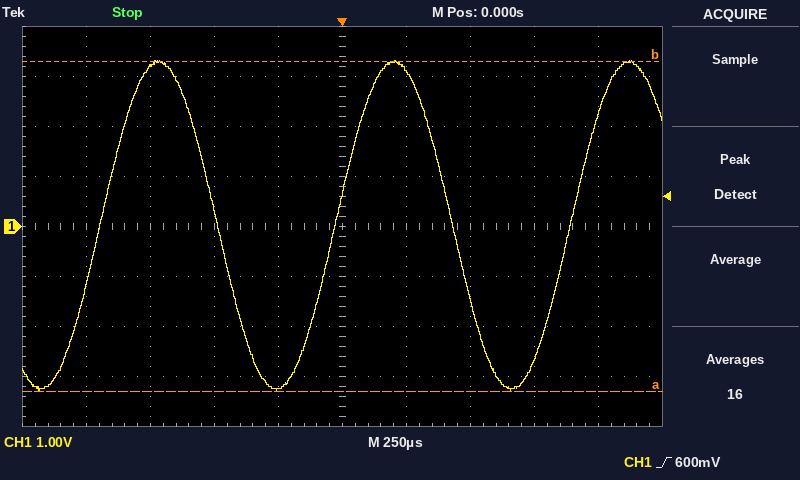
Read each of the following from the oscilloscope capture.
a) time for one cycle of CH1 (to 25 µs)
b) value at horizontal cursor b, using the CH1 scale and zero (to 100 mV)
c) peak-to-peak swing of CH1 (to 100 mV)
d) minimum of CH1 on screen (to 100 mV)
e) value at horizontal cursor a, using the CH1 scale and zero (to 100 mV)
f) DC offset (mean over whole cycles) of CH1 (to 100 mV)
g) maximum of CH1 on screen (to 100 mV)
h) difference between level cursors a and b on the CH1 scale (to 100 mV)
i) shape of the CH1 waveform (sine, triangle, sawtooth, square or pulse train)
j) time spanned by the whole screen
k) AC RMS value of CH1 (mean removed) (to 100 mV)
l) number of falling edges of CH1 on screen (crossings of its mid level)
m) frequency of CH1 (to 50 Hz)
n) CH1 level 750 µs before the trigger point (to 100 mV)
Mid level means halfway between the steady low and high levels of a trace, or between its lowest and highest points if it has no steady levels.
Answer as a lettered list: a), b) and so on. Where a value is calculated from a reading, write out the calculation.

a) 925 µs
b) 3.3 V
c) 3.3 V − (-3.3 V) = 6.6 V
d) -3.3 V
e) -3.3 V
f) (3.3 V + (-3.3 V)) / 2 ≈ 0.0 V
g) 3.3 V
h) 6.6 V
i) sine
j) 2.5 ms
k) 6.6 V / (2√2) ≈ 2.3 V
l) 2
m) 1 / 925 µs ≈ 1.08 kHz, so 1.10 kHz to the nearest 50 Hz
n) 3.2 V
